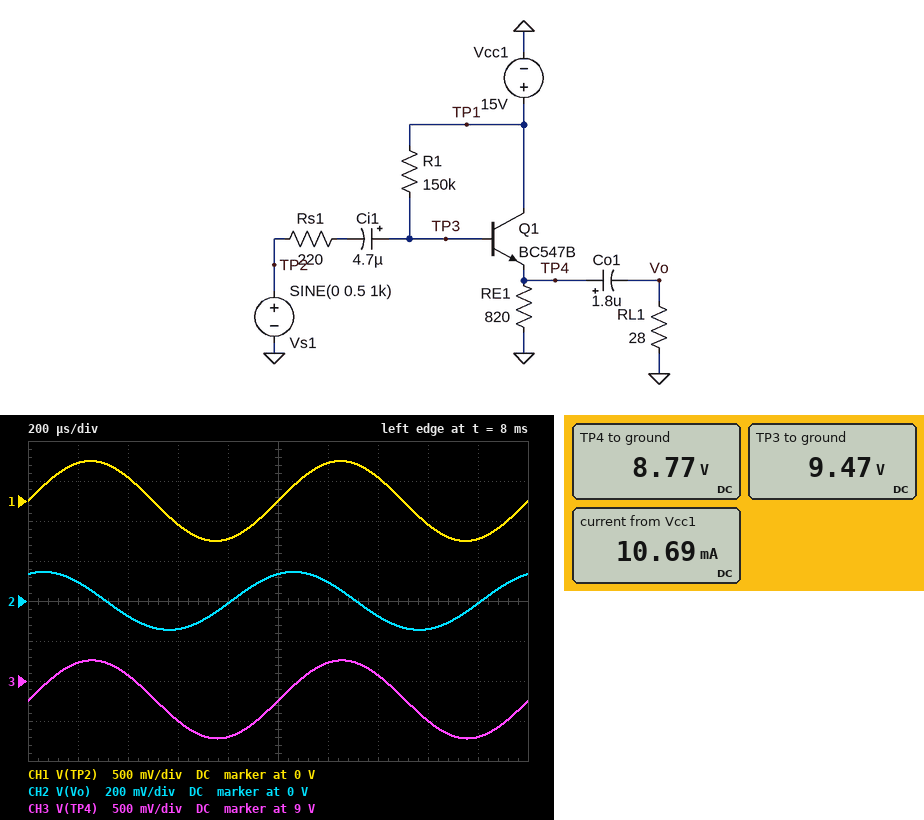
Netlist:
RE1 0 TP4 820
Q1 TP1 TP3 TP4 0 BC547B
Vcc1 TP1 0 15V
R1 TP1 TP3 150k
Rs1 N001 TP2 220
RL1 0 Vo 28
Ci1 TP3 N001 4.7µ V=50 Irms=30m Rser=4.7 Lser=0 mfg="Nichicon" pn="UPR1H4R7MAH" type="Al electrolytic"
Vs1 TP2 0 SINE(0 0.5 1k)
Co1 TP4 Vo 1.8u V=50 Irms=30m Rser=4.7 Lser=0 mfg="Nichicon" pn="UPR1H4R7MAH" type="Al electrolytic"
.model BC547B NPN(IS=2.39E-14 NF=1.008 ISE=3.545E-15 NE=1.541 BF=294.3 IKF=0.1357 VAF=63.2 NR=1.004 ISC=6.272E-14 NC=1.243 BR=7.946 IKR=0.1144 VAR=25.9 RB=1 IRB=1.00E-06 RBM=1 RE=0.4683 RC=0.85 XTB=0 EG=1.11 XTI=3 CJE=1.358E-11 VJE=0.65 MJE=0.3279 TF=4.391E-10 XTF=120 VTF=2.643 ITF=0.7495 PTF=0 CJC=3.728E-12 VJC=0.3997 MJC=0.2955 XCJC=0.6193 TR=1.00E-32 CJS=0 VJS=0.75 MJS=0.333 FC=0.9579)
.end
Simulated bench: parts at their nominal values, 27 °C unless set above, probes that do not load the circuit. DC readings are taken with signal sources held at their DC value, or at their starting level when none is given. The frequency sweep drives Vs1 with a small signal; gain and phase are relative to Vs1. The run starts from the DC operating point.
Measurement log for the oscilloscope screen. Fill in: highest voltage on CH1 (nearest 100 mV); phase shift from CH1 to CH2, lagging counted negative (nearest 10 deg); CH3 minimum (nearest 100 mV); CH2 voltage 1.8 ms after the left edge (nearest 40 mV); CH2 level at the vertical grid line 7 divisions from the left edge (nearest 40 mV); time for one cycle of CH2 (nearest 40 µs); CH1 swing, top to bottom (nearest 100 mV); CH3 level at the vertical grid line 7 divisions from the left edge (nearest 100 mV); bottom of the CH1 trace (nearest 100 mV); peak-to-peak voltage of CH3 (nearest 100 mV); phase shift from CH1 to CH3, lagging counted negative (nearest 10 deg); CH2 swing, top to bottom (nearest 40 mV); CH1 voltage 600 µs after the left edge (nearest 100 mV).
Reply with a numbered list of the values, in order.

1. 500 mV
2. 70 deg
3. 8.3 V
4. 0 V
5. -80 mV
6. 1.00 ms
7. 1.0 V
8. 9.1 V
9. -500 mV
10. 1.0 V
11. 0 deg
12. 280 mV
13. -300 mV
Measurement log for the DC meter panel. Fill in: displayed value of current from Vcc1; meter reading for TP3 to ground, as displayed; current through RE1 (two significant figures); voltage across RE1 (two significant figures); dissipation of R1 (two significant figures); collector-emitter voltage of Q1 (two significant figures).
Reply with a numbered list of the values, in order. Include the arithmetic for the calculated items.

1. 10.69 mA
2. 9.47 V
3. (8.77 V) / 820 Ω = 11 mA
4. 8.77 V = 8.8 V
5. (15 V - 9.47 V)^2 / 150 kΩ = 200 µW
6. 15 V - 8.77 V = 6.2 V
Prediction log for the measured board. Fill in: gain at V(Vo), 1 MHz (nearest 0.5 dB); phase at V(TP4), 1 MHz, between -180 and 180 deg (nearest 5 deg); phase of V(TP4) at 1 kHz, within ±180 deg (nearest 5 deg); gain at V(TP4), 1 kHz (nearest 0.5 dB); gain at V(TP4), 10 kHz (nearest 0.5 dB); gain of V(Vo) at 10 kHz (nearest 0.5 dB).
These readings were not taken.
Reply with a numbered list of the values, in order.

1. -2.5 dB
2. 0 deg
3. 0 deg
4. 0 dB
5. -1.0 dB
6. -2.5 dB
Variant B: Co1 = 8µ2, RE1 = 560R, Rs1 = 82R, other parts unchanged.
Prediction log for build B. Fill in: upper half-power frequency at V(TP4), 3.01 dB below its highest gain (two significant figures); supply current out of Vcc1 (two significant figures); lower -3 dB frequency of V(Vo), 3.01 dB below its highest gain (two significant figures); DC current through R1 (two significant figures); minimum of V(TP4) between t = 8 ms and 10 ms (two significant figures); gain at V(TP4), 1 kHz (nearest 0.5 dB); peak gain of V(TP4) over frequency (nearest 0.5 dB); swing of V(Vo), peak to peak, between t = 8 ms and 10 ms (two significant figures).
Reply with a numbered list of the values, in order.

1. 64 MHz
2. 13 mA
3. 550 Hz
4. 46 µA
5. 7.0 V
6. -0.5 dB
7. 0 dB
8. 660 mV
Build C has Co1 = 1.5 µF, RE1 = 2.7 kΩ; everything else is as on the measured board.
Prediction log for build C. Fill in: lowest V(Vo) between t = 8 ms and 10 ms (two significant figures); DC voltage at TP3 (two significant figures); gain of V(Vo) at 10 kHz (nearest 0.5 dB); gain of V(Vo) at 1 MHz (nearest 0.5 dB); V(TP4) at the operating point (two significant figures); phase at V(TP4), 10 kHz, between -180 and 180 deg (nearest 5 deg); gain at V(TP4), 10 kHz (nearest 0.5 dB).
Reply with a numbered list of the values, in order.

1. -110 mV
2. 13 V
3. -3.5 dB
4. -3.0 dB
5. 12 V
6. -5 deg
7. -1.5 dB
